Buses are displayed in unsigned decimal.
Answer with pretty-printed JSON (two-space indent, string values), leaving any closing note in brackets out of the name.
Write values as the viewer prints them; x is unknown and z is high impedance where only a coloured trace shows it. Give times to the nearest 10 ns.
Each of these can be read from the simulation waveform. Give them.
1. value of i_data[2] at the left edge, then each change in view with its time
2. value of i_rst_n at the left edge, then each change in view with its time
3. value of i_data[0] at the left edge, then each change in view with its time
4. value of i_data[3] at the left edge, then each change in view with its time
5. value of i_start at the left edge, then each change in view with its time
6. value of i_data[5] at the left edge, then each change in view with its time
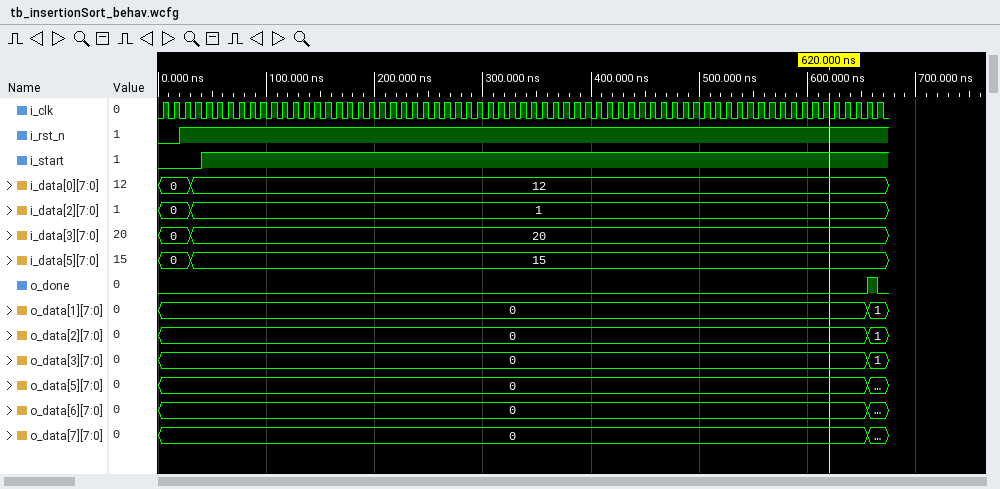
{
  "value of i_data[2] at the left edge, then each change in view with its time": "0, 1 at 30 ns",
  "value of i_rst_n at the left edge, then each change in view with its time": "0, 1 at 20 ns",
  "value of i_data[0] at the left edge, then each change in view with its time": "0, 12 at 30 ns",
  "value of i_data[3] at the left edge, then each change in view with its time": "0, 20 at 30 ns",
  "value of i_start at the left edge, then each change in view with its time": "0, 1 at 40 ns",
  "value of i_data[5] at the left edge, then each change in view with its time": "0, 15 at 30 ns"
}
